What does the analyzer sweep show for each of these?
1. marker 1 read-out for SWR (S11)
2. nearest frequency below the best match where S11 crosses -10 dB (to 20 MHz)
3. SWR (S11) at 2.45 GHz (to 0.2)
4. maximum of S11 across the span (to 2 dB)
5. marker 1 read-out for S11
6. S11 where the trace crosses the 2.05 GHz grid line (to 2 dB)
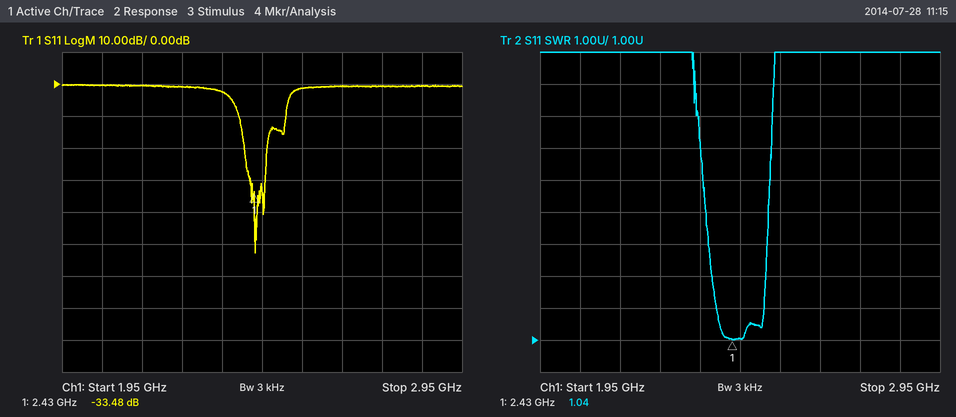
1.04
2.40 GHz
1.0
0 dB
-33.48 dB
0 dB
